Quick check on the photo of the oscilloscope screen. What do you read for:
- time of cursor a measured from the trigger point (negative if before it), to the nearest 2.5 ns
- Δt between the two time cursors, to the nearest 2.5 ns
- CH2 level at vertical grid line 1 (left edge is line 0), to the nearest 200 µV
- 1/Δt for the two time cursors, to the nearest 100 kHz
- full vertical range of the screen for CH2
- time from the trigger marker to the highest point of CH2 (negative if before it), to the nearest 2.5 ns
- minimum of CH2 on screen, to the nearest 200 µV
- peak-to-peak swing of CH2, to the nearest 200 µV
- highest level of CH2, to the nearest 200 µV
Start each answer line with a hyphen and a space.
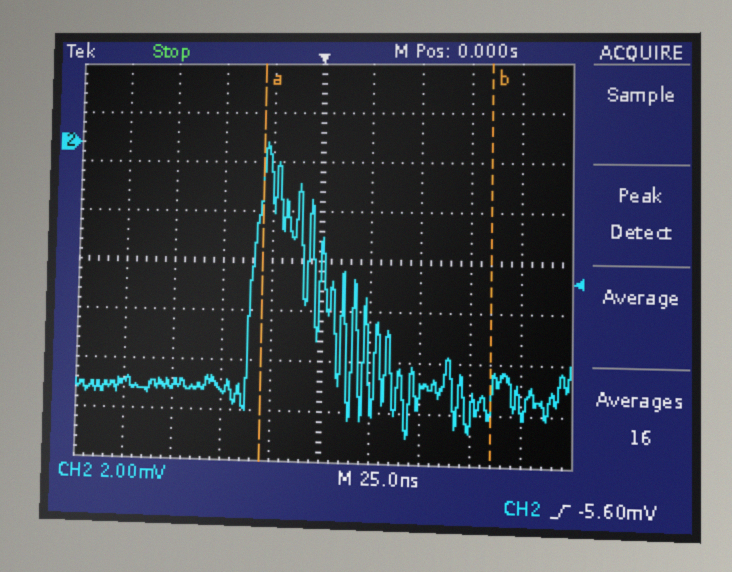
- -30.0 ns
- 115.0 ns
- -9.8 mV
- 8.7 MHz
- 16 mV
- -27.5 ns
- -11.8 mV
- 11.8 mV
- 0.0 mV
